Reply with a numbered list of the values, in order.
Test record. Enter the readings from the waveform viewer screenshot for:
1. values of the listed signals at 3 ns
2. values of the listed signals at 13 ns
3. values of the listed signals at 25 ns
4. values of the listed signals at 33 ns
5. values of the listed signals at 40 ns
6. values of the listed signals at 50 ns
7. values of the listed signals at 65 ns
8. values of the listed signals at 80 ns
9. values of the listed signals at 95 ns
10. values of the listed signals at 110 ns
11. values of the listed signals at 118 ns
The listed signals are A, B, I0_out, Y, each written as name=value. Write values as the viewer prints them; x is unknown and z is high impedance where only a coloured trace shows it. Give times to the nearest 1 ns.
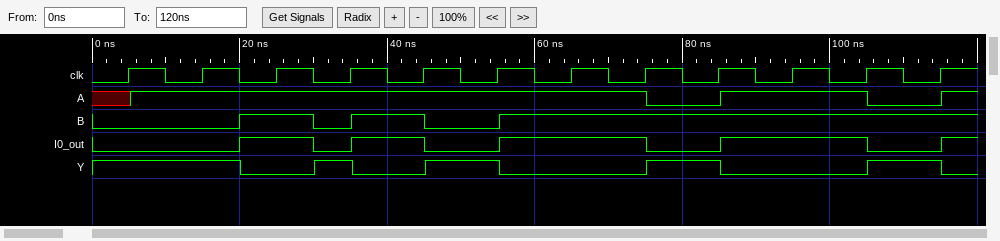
1. A=x, B=0, I0_out=0, Y=1
2. A=1, B=0, I0_out=0, Y=1
3. A=1, B=1, I0_out=1, Y=0
4. A=1, B=0, I0_out=0, Y=1
5. A=1, B=1, I0_out=1, Y=0
6. A=1, B=0, I0_out=0, Y=1
7. A=1, B=1, I0_out=1, Y=0
8. A=0, B=1, I0_out=0, Y=1
9. A=1, B=1, I0_out=1, Y=0
10. A=0, B=1, I0_out=0, Y=1
11. A=1, B=1, I0_out=1, Y=0
